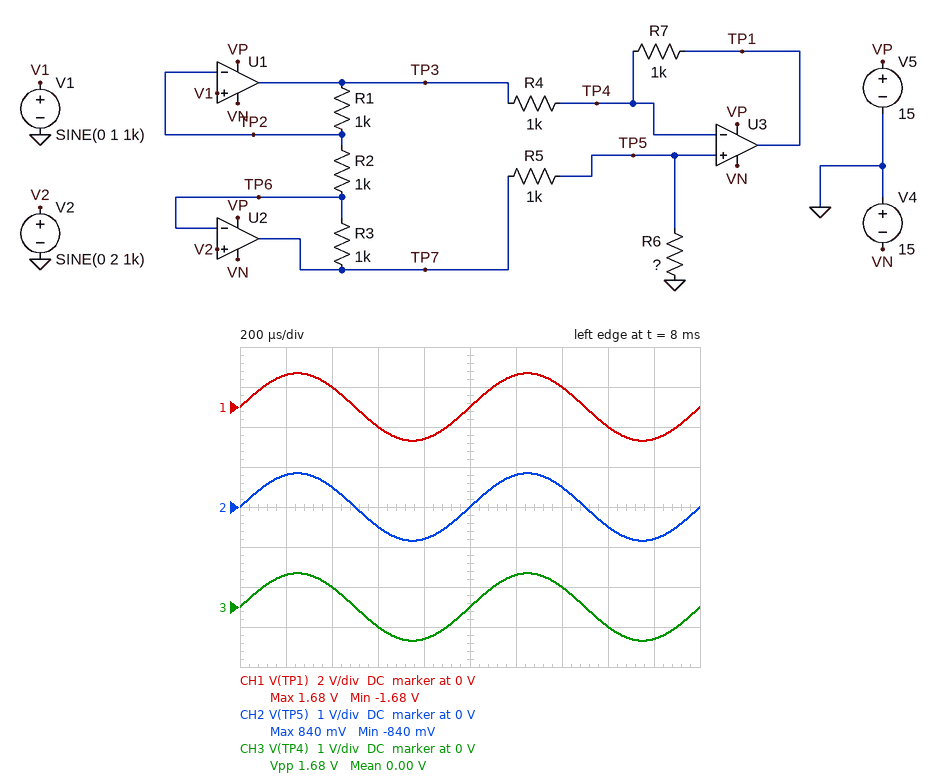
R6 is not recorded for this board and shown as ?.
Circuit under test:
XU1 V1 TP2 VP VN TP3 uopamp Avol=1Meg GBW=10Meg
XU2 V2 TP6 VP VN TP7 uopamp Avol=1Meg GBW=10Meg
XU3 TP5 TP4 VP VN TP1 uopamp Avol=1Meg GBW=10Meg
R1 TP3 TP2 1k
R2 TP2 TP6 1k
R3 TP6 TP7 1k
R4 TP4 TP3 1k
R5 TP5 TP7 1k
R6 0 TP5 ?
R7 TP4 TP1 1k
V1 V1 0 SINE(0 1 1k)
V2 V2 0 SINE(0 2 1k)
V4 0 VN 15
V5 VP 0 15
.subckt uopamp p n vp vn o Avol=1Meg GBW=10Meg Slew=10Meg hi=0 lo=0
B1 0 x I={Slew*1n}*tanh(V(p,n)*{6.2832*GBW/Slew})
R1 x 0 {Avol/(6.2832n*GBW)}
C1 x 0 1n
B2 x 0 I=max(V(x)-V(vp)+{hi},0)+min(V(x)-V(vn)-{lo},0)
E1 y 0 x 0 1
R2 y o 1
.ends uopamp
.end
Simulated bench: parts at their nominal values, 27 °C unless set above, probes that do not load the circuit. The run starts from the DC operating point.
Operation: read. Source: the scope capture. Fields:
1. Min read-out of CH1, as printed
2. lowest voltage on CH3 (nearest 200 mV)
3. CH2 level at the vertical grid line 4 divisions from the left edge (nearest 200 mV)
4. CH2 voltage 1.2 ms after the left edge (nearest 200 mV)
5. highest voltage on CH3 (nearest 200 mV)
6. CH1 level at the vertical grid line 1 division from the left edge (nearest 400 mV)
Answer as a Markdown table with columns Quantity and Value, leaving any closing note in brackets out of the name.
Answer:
| Quantity | Value |
|---|---|
| Min read-out of CH1, as printed | -1.68 V |
| lowest voltage on CH3 | -800 mV |
| CH2 level at the vertical grid line 4 divisions from the left edge | -800 mV |
| CH2 voltage 1.2 ms after the left edge | 800 mV |
| highest voltage on CH3 | 800 mV |
| CH1 level at the vertical grid line 1 division from the left edge | 1.6 V |
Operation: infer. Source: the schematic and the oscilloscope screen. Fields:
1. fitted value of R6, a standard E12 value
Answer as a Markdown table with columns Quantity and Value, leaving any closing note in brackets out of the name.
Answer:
| Quantity | Value |
|---|---|
| fitted value of R6, a standard E12 value | 390 Ω |
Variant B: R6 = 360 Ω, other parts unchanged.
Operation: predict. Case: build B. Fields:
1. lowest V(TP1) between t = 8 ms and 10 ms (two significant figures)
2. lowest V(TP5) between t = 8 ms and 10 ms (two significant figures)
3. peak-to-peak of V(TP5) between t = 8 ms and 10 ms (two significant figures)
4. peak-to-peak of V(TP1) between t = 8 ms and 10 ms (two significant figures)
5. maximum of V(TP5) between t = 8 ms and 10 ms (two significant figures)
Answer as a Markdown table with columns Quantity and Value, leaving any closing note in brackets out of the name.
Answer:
| Quantity | Value |
|---|---|
| lowest V(TP1) between t = 8 ms and 10 ms | -1.6 V |
| lowest V(TP5) between t = 8 ms and 10 ms | -790 mV |
| peak-to-peak of V(TP5) between t = 8 ms and 10 ms | 1.6 V |
| peak-to-peak of V(TP1) between t = 8 ms and 10 ms | 3.2 V |
| maximum of V(TP5) between t = 8 ms and 10 ms | 790 mV |
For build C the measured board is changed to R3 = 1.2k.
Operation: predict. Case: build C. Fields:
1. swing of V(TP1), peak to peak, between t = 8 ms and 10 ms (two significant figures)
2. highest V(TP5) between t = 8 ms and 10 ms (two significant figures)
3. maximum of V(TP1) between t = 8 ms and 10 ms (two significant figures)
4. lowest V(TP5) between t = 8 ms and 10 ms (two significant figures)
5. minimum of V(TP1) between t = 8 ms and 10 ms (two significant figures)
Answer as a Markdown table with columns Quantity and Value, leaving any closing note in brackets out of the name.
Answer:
| Quantity | Value |
|---|---|
| swing of V(TP1), peak to peak, between t = 8 ms and 10 ms | 3.6 V |
| highest V(TP5) between t = 8 ms and 10 ms | 900 mV |
| maximum of V(TP1) between t = 8 ms and 10 ms | 1.8 V |
| lowest V(TP5) between t = 8 ms and 10 ms | -900 mV |
| minimum of V(TP1) between t = 8 ms and 10 ms | -1.8 V |
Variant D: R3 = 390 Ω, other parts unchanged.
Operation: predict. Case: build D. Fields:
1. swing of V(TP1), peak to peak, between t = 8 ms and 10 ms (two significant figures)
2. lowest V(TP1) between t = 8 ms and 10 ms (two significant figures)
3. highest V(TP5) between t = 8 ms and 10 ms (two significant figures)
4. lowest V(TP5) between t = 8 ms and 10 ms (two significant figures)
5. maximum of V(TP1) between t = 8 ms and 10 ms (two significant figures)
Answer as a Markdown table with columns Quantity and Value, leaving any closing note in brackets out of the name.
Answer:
| Quantity | Value |
|---|---|
| swing of V(TP1), peak to peak, between t = 8 ms and 10 ms | 2.7 V |
| lowest V(TP1) between t = 8 ms and 10 ms | -1.3 V |
| highest V(TP5) between t = 8 ms and 10 ms | 670 mV |
| lowest V(TP5) between t = 8 ms and 10 ms | -670 mV |
| maximum of V(TP1) between t = 8 ms and 10 ms | 1.3 V |
